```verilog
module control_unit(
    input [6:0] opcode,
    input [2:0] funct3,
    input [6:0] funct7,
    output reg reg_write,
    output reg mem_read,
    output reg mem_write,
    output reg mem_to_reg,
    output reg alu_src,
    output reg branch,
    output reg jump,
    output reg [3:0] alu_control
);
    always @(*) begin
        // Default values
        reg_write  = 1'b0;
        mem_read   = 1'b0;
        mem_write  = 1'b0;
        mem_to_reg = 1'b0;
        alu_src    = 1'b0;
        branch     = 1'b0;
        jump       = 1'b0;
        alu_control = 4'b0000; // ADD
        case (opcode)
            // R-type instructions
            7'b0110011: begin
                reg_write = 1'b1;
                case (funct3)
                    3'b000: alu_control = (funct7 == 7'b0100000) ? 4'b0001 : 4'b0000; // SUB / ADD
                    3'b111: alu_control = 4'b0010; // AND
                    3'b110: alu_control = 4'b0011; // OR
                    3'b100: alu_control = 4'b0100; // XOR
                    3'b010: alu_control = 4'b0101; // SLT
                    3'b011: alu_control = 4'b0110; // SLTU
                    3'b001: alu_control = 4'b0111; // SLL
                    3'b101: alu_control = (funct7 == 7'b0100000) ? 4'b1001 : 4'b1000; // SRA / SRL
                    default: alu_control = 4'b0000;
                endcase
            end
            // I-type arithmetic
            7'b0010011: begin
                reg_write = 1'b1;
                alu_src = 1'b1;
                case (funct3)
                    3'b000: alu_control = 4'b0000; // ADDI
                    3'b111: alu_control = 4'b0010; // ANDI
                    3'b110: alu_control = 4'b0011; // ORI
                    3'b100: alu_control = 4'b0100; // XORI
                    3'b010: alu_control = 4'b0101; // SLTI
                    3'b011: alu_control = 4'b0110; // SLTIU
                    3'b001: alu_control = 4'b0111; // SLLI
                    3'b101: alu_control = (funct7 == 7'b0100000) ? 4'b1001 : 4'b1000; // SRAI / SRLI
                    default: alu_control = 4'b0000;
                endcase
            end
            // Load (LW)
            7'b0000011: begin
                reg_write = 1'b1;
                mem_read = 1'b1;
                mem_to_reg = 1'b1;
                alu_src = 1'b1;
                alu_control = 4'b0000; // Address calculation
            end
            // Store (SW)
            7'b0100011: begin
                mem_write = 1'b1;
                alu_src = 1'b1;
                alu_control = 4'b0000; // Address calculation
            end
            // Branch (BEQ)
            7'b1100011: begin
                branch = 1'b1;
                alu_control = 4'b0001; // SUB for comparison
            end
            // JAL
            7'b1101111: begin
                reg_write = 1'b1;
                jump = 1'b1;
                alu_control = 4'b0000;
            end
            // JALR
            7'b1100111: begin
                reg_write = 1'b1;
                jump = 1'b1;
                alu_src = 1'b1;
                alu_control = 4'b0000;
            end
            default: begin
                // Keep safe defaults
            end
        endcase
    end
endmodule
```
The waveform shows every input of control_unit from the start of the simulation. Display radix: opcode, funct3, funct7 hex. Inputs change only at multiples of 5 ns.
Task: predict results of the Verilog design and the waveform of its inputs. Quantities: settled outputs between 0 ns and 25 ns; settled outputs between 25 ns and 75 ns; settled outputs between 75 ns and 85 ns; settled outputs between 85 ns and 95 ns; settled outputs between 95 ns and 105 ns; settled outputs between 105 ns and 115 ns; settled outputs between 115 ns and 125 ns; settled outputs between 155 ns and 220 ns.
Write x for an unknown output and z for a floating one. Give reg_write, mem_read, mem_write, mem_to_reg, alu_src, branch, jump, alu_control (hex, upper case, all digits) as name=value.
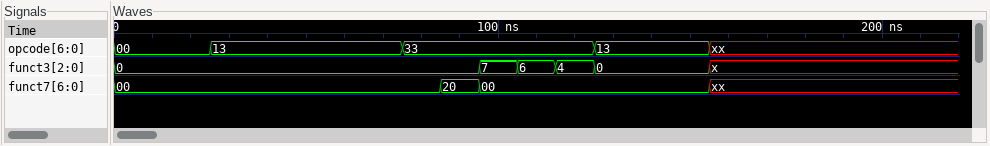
reg_write=0, mem_read=0, mem_write=0, mem_to_reg=0, alu_src=0, branch=0, jump=0, alu_control=0
reg_write=1, mem_read=0, mem_write=0, mem_to_reg=0, alu_src=1, branch=0, jump=0, alu_control=0
reg_write=1, mem_read=0, mem_write=0, mem_to_reg=0, alu_src=0, branch=0, jump=0, alu_control=0
reg_write=1, mem_read=0, mem_write=0, mem_to_reg=0, alu_src=0, branch=0, jump=0, alu_control=1
reg_write=1, mem_read=0, mem_write=0, mem_to_reg=0, alu_src=0, branch=0, jump=0, alu_control=2
reg_write=1, mem_read=0, mem_write=0, mem_to_reg=0, alu_src=0, branch=0, jump=0, alu_control=3
reg_write=1, mem_read=0, mem_write=0, mem_to_reg=0, alu_src=0, branch=0, jump=0, alu_control=4
reg_write=0, mem_read=0, mem_write=0, mem_to_reg=0, alu_src=0, branch=0, jump=0, alu_control=0
